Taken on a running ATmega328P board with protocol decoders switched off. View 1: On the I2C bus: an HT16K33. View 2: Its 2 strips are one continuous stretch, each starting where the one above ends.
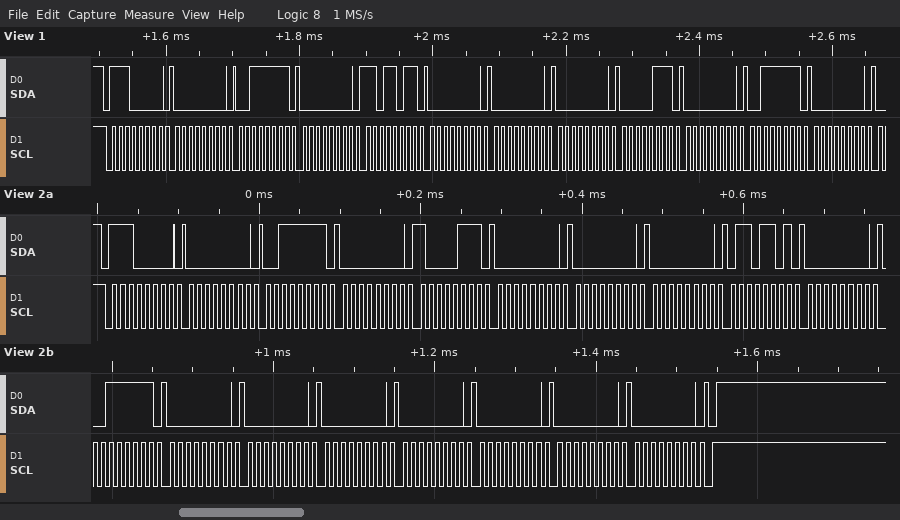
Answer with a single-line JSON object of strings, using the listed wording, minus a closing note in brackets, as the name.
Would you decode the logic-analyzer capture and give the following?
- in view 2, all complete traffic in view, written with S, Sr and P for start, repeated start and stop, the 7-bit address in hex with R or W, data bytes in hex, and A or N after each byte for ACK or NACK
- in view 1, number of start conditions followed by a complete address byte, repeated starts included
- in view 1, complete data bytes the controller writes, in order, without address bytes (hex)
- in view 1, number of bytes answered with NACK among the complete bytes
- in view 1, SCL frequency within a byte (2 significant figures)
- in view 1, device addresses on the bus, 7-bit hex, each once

{"in view 2, all complete traffic in view, written with S, Sr and P for start, repeated start and stop, the 7-bit address in hex with R or W, data bytes in hex, and A or N after each byte for ACK or NACK": "S 70W A 00 A 3F A 00 A 87 A 00 A 00 A 00 A 6D A 00 A 3F A 00 A 00 A 00 A 00 A 00 A 00 A 00 A P", "in view 1, number of start conditions followed by a complete address byte, repeated starts included": "1", "in view 1, complete data bytes the controller writes, in order, without address bytes": "00 3F 00 DB 00 00 00 07 00 3F 00", "in view 1, number of bytes answered with NACK among the complete bytes": "0", "in view 1, SCL frequency within a byte": "100 kHz", "in view 1, device addresses on the bus, 7-bit hex, each once": "0x70"}
